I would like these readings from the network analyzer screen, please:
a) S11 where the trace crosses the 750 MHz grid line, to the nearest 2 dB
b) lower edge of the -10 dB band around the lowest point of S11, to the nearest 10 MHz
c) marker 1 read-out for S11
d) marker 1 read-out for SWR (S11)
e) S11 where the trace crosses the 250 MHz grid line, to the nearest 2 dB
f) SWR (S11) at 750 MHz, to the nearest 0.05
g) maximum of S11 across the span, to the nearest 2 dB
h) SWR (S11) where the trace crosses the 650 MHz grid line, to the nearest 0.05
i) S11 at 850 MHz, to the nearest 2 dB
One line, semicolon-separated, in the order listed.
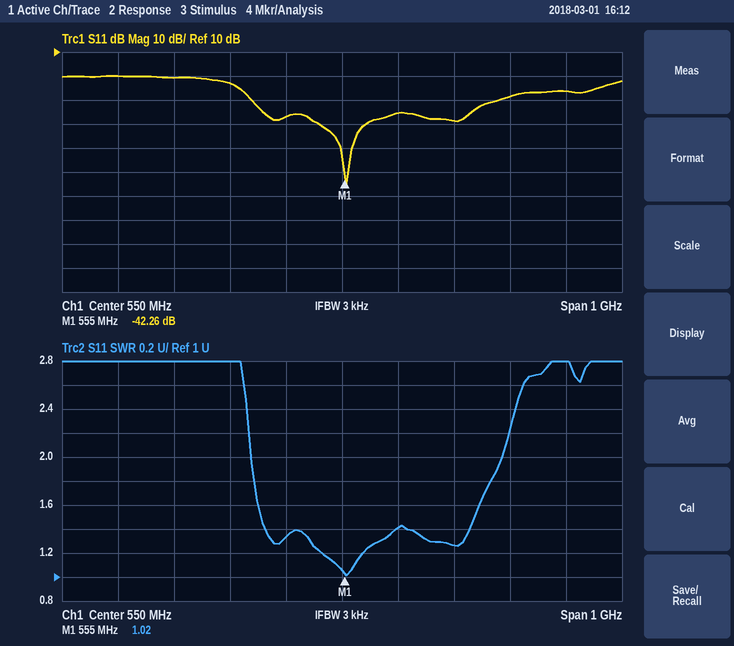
-18 dB; 390 MHz; -42.26 dB; 1.02; 0 dB; 1.25; 0 dB; 1.40; -8 dB
